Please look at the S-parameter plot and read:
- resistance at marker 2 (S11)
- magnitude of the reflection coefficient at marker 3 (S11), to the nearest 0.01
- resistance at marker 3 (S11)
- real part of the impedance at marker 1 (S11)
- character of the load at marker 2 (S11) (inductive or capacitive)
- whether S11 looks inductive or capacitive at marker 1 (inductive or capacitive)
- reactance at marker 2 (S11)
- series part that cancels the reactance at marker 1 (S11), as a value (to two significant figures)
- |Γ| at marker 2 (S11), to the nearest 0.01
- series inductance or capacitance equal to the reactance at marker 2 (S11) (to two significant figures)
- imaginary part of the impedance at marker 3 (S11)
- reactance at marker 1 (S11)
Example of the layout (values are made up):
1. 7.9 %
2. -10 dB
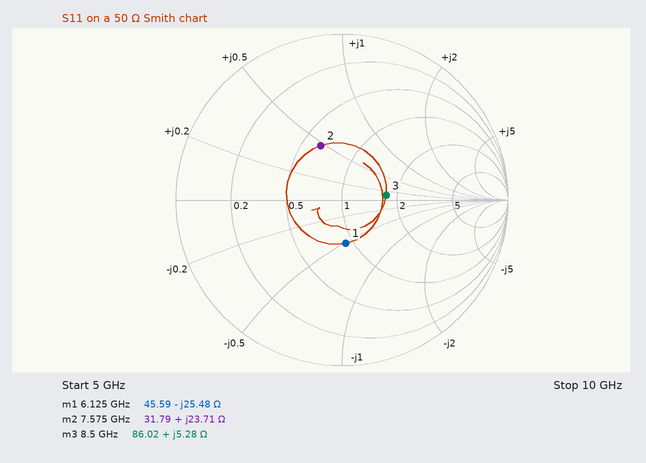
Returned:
1. 31.79 Ω
2. 0.27
3. 86.02 Ω
4. 45.59 Ω
5. inductive
6. capacitive
7. +23.71 Ω
8. 660 pH
9. 0.35
10. 500 pH
11. +5.28 Ω
12. -25.48 Ω
